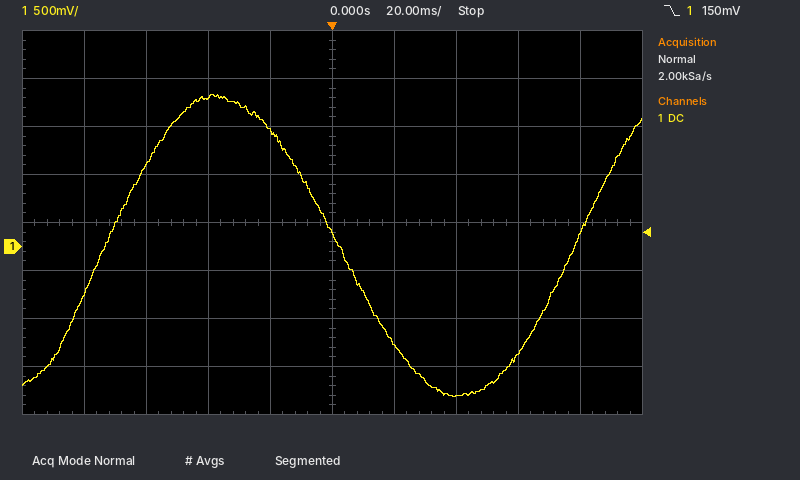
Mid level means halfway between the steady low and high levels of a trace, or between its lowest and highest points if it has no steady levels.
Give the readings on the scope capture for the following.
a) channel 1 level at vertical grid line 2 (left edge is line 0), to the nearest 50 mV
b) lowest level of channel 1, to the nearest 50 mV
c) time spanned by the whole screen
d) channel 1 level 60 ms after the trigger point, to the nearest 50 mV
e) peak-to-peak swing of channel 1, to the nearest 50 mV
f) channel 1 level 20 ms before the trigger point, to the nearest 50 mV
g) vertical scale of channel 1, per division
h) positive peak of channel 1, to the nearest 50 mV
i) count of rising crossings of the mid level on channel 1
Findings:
850 mV
-1.55 V
200 ms
-1.10 V
3.15 V
1.20 V
500 mV
1.60 V
2
